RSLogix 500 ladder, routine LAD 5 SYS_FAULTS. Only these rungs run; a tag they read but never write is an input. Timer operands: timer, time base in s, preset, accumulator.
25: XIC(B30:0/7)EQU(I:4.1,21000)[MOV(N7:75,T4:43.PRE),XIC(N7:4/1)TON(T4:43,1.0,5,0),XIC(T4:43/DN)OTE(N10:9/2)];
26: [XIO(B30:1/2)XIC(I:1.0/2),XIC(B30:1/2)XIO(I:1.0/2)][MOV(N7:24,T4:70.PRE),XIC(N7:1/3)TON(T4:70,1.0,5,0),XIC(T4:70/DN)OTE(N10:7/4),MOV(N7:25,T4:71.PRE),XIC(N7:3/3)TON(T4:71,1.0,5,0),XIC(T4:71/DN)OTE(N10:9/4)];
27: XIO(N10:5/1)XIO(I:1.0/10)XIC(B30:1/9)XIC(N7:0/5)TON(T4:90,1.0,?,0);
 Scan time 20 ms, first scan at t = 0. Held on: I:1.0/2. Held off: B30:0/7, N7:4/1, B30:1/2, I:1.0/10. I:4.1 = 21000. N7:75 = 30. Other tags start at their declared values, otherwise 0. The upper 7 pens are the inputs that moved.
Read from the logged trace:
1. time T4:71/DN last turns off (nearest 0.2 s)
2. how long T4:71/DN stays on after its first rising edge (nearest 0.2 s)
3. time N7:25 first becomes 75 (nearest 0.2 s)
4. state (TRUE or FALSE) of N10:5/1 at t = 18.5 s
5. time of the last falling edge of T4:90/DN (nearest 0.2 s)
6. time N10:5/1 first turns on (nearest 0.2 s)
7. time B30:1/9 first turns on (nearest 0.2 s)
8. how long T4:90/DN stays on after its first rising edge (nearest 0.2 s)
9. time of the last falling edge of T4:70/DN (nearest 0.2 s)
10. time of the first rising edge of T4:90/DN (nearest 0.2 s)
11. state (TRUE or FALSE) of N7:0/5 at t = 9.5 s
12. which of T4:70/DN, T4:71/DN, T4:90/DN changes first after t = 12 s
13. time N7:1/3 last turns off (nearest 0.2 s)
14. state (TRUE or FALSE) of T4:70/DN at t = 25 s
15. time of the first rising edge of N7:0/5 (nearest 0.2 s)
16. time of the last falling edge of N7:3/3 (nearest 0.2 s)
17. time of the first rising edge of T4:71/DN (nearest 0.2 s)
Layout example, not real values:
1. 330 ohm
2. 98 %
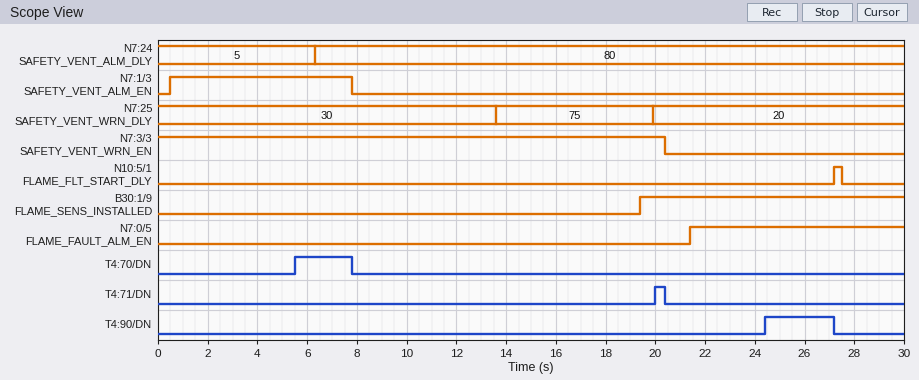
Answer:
1. 20.4 s
2. 0.4 s
3. 13.6 s
4. FALSE
5. 27.2 s
6. 27.2 s
7. 19.4 s
8. 2.8 s
9. 7.8 s
10. 24.4 s
11. FALSE
12. T4:71/DN
13. 7.8 s
14. FALSE
15. 21.4 s
16. 20.4 s
17. 20.0 s
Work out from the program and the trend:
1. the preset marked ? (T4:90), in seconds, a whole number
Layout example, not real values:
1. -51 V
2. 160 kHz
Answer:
1. 3 s
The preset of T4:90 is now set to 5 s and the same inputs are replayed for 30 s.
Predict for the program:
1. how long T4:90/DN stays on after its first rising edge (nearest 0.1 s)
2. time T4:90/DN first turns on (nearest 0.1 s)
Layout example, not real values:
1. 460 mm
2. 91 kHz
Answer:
1. 0.8 s
2. 26.4 s
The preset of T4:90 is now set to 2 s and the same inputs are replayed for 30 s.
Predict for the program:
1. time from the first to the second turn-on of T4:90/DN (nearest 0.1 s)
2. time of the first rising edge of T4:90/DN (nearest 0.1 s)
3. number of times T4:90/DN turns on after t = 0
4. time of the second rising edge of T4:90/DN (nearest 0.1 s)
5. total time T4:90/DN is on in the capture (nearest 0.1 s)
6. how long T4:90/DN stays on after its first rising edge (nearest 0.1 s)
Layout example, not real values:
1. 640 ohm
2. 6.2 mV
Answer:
1. 6.1 s
2. 23.4 s
3. 2
4. 29.5 s
5. 4.3 s
6. 3.8 s
